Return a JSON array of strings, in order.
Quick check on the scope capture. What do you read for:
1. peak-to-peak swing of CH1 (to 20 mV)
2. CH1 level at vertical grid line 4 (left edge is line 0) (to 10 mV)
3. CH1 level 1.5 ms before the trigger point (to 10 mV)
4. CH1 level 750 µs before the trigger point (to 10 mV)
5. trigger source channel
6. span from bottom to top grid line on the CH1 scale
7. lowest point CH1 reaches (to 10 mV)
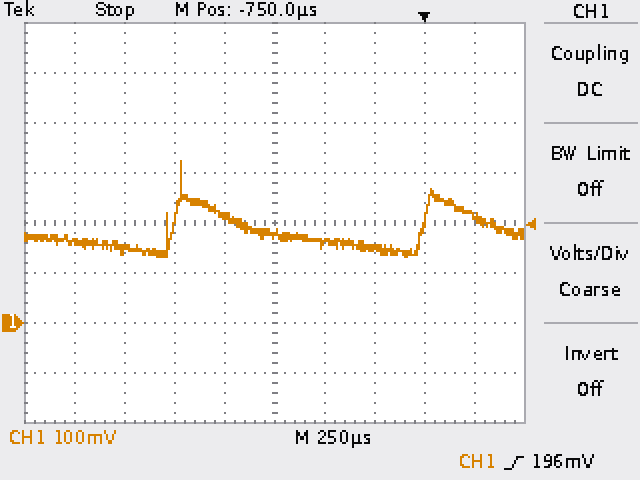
["200 mV", "210 mV", "150 mV", "180 mV", "CH1", "800 mV", "130 mV"]
